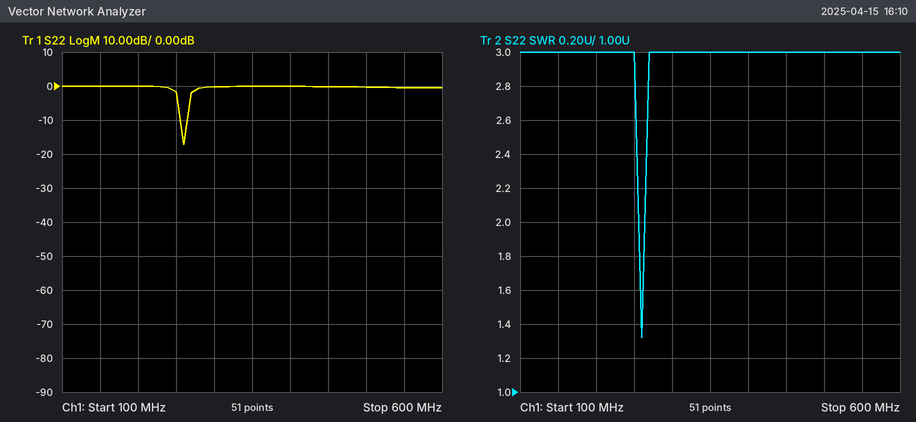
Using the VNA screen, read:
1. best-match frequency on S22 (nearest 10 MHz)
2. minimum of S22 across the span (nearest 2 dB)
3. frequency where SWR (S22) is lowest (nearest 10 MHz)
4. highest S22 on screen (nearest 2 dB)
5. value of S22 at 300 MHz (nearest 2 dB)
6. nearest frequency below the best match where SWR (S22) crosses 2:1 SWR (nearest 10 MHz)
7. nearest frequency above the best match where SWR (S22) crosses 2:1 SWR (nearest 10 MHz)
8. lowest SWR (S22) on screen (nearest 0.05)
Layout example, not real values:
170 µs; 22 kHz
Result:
260 MHz; -18 dB; 260 MHz; 0 dB; 0 dB; 260 MHz; 260 MHz; 1.30
